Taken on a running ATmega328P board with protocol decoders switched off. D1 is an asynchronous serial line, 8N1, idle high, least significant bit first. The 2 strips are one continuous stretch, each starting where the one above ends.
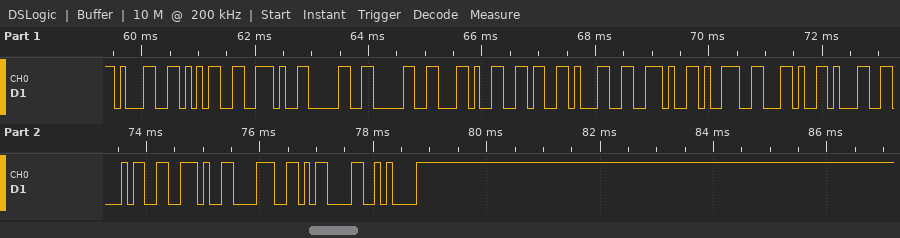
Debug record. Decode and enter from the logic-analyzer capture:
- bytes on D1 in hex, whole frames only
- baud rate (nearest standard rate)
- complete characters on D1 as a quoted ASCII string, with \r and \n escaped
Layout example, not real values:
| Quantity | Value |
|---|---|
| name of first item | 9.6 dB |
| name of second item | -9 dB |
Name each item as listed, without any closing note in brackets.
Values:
| Quantity | Value |
|---|---|
| bytes on D1 in hex, whole frames only | 31 35 2E 30 30 2C 36 31 2E 39 2C 31 34 2E 38 0D 0A |
| baud rate | 9600 baud |
| complete characters on D1 as a quoted ASCII string, with \r and \n escaped | "15.00,61.9,14.8\r\n" |
